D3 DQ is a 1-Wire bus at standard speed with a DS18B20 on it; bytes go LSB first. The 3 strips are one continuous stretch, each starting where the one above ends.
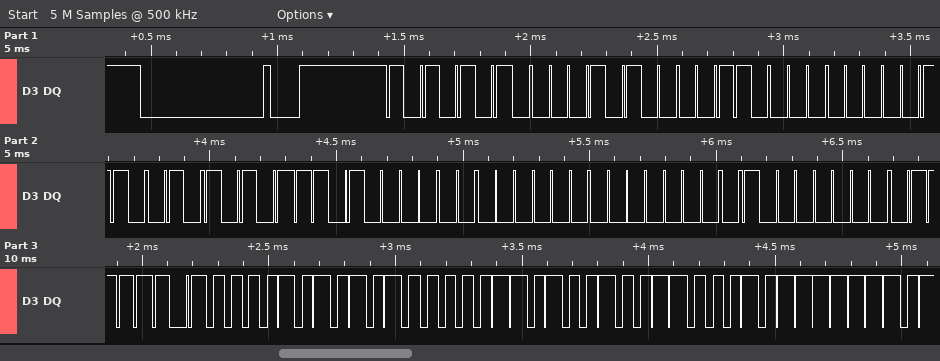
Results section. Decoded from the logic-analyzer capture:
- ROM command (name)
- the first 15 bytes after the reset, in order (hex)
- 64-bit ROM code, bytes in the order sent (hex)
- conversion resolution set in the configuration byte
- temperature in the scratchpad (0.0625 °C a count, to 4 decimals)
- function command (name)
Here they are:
Match ROM
55 28 0C 60 AA 0B 00 00 01 BE 50 05 4B 46 7F
28 0C 60 AA 0B 00 00 01
12 bits
85.0000 °C
Read Scratchpad
